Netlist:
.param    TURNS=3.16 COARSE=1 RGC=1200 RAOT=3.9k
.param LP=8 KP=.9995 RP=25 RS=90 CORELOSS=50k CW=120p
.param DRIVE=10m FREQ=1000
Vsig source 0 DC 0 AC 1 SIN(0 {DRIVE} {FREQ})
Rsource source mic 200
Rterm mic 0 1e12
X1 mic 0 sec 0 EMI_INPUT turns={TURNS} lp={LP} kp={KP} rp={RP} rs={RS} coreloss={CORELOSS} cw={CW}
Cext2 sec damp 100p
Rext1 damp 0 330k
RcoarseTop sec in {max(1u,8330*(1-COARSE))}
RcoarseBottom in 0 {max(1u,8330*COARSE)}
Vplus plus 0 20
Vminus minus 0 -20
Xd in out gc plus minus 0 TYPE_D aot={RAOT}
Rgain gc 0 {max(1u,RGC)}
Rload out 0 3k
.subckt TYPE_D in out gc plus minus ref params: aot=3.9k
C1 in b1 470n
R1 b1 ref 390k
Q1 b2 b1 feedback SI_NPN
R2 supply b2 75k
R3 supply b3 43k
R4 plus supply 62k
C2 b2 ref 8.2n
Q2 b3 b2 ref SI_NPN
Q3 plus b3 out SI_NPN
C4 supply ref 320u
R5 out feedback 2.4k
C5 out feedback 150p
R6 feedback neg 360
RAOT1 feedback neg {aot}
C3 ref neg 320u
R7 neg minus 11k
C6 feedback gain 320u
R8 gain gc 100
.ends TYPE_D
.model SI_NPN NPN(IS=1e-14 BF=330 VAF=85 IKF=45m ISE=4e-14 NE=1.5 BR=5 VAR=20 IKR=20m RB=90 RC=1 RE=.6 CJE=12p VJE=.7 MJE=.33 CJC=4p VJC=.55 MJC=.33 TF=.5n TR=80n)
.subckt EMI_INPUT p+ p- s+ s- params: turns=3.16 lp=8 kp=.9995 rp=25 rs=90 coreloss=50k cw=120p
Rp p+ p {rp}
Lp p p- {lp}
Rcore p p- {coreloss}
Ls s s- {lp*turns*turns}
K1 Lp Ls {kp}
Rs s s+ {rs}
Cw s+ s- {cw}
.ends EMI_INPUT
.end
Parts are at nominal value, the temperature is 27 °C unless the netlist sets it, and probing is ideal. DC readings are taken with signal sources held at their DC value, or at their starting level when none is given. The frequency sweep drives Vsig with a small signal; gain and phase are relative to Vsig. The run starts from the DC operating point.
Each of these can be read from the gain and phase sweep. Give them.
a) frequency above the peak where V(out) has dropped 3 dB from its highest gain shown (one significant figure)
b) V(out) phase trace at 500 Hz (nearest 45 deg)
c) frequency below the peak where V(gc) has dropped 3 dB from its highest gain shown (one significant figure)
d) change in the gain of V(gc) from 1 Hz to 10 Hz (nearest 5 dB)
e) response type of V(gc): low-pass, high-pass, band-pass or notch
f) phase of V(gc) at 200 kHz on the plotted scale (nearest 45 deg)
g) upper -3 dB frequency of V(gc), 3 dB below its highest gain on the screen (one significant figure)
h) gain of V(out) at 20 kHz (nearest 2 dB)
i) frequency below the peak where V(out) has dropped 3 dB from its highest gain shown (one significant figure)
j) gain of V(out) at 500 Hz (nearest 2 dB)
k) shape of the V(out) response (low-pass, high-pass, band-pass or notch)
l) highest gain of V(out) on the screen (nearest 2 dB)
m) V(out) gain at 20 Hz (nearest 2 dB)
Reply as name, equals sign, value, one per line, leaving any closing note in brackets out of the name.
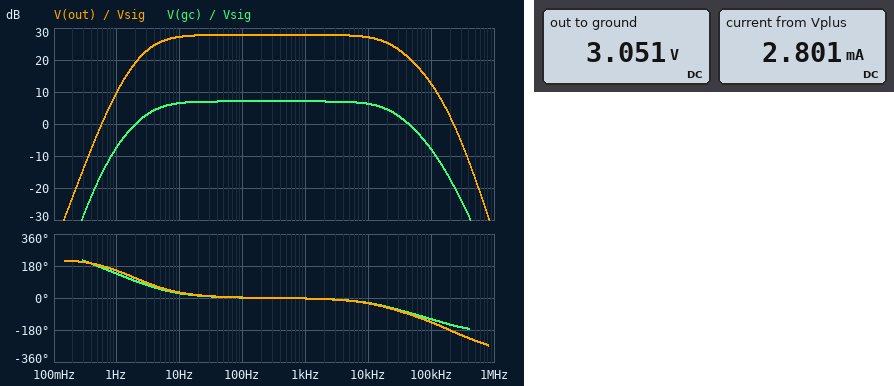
frequency above the peak where V(out) has dropped 3 dB from its highest gain shown = 20 kHz
V(out) phase trace at 500 Hz = 0 deg
frequency below the peak where V(gc) has dropped 3 dB from its highest gain shown = 4 Hz
change in the gain of V(gc) from 1 Hz to 10 Hz = 15 dB
response type of V(gc): low-pass, high-pass, band-pass or notch = band-pass
phase of V(gc) at 200 kHz on the plotted scale = -135 deg
upper -3 dB frequency of V(gc), 3 dB below its highest gain on the screen = 20 kHz
gain of V(out) at 20 kHz = 26 dB
frequency below the peak where V(out) has dropped 3 dB from its highest gain shown = 4 Hz
gain of V(out) at 500 Hz = 28 dB
shape of the V(out) response = band-pass
highest gain of V(out) on the screen = 28 dB
V(out) gain at 20 Hz = 28 dB
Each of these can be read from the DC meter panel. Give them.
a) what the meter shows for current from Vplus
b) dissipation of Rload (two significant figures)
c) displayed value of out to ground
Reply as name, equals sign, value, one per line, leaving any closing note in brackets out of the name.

what the meter shows for current from Vplus = 2.801 mA
dissipation of Rload = 3.1 mW
displayed value of out to ground = 3.051 V
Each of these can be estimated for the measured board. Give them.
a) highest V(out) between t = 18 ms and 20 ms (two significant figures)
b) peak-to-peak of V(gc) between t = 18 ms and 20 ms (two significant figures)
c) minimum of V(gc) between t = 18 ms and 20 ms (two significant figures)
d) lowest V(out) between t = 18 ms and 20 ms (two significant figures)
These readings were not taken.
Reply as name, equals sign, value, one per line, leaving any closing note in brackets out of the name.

highest V(out) between t = 18 ms and 20 ms = 3.3 V
peak-to-peak of V(gc) between t = 18 ms and 20 ms = 45 mV
minimum of V(gc) between t = 18 ms and 20 ms = -23 mV
lowest V(out) between t = 18 ms and 20 ms = 2.8 V
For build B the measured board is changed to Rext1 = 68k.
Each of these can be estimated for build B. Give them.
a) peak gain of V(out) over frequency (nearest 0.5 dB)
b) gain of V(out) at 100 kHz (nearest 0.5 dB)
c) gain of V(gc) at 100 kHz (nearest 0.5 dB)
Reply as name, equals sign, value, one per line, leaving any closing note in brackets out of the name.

peak gain of V(out) over frequency = 28.0 dB
gain of V(out) at 100 kHz = 12.0 dB
gain of V(gc) at 100 kHz = -8.5 dB
